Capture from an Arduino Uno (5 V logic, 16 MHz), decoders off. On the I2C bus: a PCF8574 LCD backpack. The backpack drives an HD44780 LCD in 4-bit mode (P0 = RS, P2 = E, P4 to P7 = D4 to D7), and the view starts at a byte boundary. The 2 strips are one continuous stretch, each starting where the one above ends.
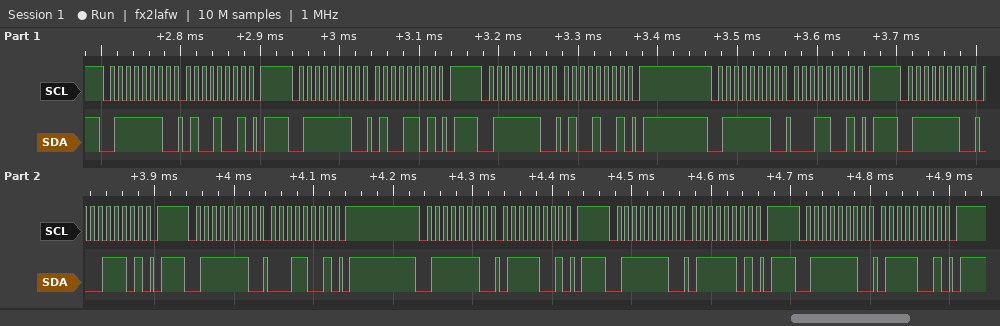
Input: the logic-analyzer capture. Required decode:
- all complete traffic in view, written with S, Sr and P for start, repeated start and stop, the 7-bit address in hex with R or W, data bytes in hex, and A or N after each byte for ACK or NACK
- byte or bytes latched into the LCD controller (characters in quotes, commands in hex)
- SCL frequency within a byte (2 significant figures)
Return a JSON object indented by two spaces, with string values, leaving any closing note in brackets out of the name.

{
  "all complete traffic in view, written with S, Sr and P for start, repeated start and stop, the 7-bit address in hex with R or W, data bytes in hex, and A or N after each byte for ACK or NACK": "S 3FW A 49 A P S 3FW A 4D A P S 3FW A 49 A P S 3FW A 19 A P S 3FW A 1D A P S 3FW A 19 A P S 3FW A 79 A P S 3FW A 7D A P S 3FW A 79 A P",
  "byte or bytes latched into the LCD controller": "'A'",
  "SCL frequency within a byte": "100 kHz"
}
